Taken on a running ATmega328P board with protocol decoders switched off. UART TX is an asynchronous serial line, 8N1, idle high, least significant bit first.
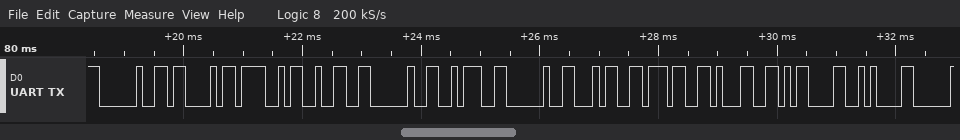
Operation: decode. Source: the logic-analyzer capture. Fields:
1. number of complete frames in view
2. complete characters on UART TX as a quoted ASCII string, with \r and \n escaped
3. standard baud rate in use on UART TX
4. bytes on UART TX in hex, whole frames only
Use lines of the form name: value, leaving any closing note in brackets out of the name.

number of complete frames in view: 12
complete characters on UART TX as a quoted ASCII string, with \r and \n escaped: " CO2 : 471\r\n"
standard baud rate in use on UART TX: 9600 baud
bytes on UART TX in hex, whole frames only: 0x20 0x43 0x4F 0x32 0x20 0x3A 0x20 0x34 0x37 0x31 0x0D 0x0A
